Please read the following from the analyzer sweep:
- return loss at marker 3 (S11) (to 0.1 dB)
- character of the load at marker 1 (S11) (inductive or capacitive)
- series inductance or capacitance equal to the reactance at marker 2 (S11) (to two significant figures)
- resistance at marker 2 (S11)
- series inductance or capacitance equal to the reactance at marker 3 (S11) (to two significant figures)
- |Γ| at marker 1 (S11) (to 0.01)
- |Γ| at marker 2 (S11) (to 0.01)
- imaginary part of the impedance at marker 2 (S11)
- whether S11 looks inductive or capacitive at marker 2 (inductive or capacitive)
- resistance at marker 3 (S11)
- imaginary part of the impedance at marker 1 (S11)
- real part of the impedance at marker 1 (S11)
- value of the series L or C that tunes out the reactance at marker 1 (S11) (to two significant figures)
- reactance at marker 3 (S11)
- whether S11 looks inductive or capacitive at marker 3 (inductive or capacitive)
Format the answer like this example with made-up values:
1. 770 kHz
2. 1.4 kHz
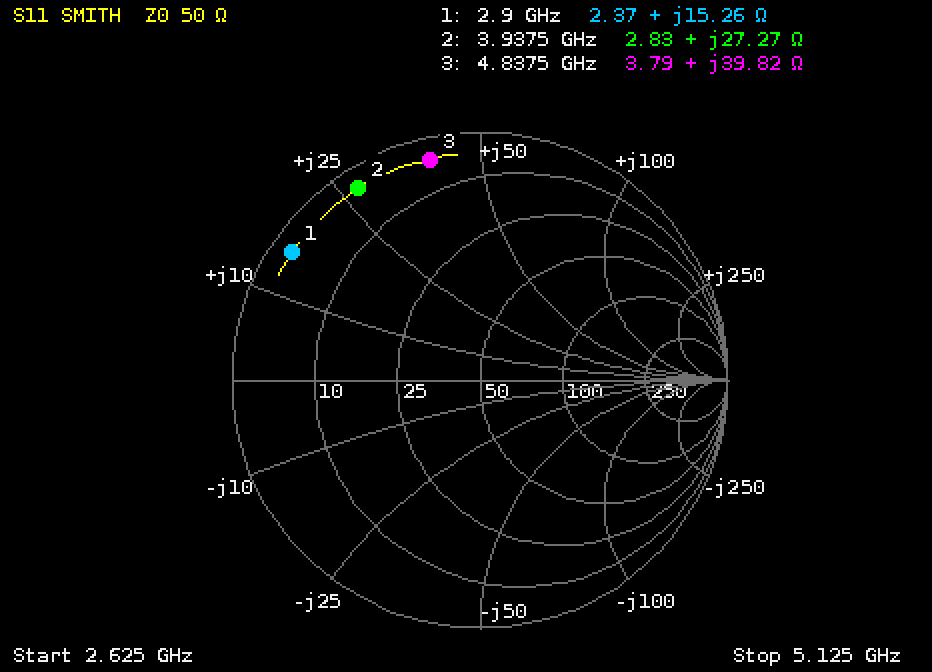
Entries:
1. 0.8 dB
2. inductive
3. 1.1 nH
4. 2.83 Ω
5. 1.3 nH
6. 0.92
7. 0.92
8. +27.27 Ω
9. inductive
10. 3.79 Ω
11. +15.26 Ω
12. 2.37 Ω
13. 3.6 pF
14. +39.82 Ω
15. inductive
